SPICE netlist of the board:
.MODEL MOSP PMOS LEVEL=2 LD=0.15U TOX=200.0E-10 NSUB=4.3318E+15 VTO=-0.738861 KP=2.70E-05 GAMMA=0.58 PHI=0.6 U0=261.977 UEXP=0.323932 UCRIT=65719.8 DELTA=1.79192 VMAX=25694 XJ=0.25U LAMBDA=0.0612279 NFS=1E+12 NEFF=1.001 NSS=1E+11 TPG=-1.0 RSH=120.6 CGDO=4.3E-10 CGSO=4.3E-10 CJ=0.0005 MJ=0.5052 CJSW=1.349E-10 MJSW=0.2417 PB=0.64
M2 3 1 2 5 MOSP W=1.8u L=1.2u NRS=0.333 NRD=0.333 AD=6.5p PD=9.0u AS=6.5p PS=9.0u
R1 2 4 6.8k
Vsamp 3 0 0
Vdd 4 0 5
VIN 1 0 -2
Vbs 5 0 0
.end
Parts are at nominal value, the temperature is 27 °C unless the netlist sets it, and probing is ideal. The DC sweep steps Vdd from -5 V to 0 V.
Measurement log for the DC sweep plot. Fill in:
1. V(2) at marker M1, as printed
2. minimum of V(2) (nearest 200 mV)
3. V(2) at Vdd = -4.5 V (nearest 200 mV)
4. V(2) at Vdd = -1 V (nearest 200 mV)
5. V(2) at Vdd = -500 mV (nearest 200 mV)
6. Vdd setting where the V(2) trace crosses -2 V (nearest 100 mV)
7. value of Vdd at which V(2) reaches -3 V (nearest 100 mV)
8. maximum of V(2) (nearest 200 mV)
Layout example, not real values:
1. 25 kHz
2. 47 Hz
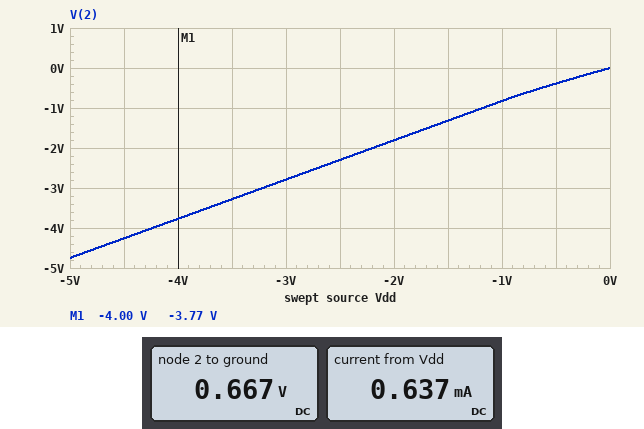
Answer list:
1. -3.77 V
2. -4.8 V
3. -4.2 V
4. -800 mV
5. -400 mV
6. -2.2 V
7. -3.2 V
8. 0 V
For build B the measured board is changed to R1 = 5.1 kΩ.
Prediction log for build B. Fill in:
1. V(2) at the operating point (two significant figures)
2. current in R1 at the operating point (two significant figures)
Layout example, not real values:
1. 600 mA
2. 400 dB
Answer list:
1. 680 mV
2. 850 µA
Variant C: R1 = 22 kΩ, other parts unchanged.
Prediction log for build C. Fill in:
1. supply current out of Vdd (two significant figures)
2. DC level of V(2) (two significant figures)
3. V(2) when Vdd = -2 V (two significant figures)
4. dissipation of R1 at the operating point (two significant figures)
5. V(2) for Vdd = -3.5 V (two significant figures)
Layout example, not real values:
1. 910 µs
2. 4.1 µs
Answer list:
1. 200 µA
2. 620 mV
3. -1.4 V
4. 870 µW
5. -2.8 V
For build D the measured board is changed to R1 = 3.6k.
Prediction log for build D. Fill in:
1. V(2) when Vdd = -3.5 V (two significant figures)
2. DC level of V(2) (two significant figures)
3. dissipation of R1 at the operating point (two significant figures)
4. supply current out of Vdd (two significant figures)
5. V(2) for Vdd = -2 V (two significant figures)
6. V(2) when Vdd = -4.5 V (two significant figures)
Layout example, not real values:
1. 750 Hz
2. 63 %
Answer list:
1. -3.4 V
2. 710 mV
3. 5.1 mW
4. 1.2 mA
5. -1.9 V
6. -4.4 V
